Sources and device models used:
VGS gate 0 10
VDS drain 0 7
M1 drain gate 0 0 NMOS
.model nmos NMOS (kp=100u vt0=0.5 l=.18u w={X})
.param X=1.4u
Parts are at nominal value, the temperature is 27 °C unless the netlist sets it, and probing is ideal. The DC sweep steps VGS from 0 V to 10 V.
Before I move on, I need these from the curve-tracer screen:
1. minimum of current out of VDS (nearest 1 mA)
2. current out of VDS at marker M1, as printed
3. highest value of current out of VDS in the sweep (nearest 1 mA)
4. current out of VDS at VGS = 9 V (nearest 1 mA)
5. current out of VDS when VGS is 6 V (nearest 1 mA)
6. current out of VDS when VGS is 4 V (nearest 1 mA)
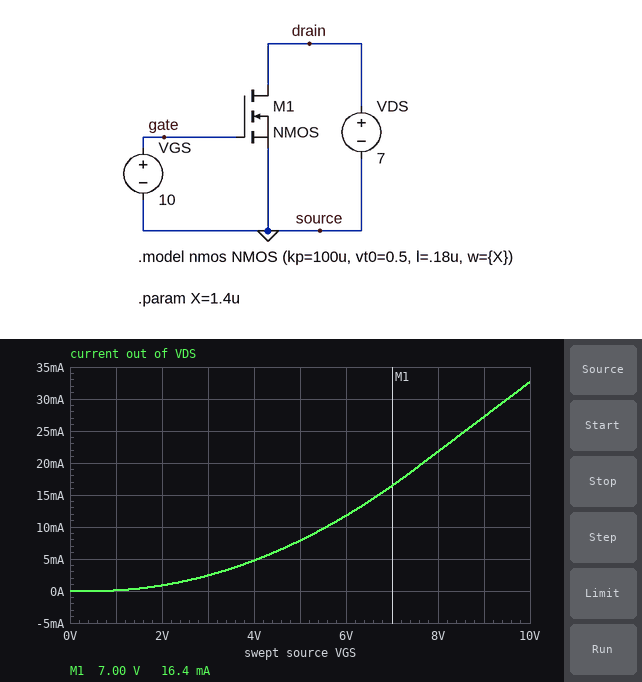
0 A
16.4 mA
33 mA
27 mA
12 mA
5 mA
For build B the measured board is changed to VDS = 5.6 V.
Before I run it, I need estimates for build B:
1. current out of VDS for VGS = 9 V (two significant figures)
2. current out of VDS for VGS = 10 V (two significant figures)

25 mA
29 mA
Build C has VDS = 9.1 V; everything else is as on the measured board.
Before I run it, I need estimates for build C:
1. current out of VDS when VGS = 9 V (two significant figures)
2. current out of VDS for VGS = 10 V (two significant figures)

28 mA
35 mA
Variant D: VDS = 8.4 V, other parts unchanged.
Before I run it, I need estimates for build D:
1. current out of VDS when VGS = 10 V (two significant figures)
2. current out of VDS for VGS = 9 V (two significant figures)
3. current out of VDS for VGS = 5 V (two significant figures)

35 mA
28 mA
7.9 mA
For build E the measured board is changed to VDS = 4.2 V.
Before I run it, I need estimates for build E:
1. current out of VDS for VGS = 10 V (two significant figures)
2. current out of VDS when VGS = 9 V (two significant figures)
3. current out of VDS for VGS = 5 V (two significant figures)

24 mA
21 mA
7.8 mA
